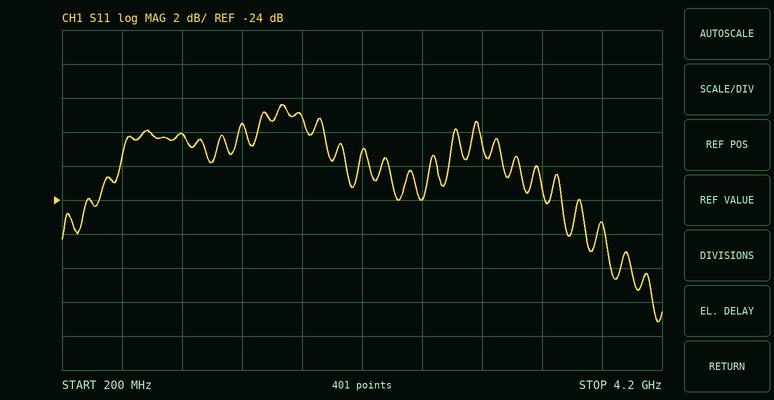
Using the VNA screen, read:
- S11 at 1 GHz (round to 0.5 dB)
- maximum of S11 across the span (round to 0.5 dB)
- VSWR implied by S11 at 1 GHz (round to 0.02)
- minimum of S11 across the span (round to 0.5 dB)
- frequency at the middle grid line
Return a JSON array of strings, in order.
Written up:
["-20.0 dB", "-18.5 dB", "1.22", "-31.0 dB", "2.2 GHz"]
